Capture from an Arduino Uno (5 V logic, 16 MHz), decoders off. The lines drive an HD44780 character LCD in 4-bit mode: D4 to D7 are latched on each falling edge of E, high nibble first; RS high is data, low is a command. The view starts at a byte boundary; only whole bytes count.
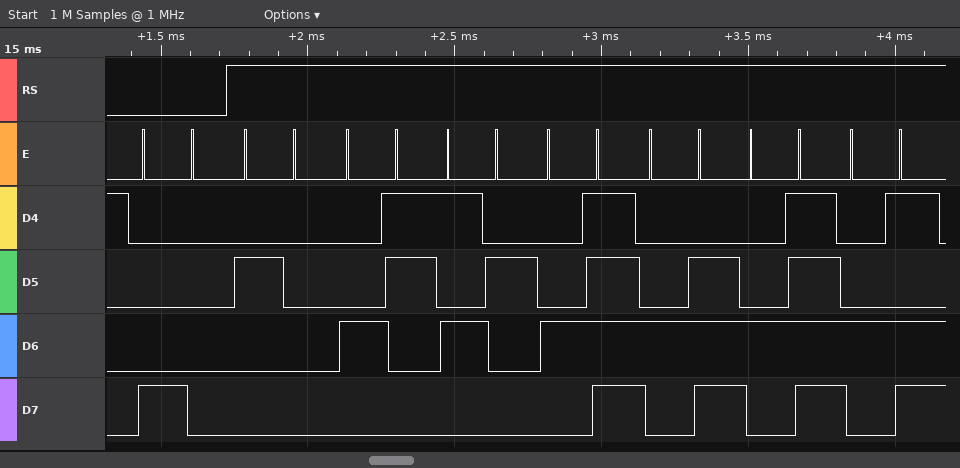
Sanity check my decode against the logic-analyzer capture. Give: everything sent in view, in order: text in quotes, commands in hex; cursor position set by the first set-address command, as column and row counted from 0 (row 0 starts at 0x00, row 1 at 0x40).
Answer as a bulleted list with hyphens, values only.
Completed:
- 0x80 " CRONOM"
- column 0, row 0
